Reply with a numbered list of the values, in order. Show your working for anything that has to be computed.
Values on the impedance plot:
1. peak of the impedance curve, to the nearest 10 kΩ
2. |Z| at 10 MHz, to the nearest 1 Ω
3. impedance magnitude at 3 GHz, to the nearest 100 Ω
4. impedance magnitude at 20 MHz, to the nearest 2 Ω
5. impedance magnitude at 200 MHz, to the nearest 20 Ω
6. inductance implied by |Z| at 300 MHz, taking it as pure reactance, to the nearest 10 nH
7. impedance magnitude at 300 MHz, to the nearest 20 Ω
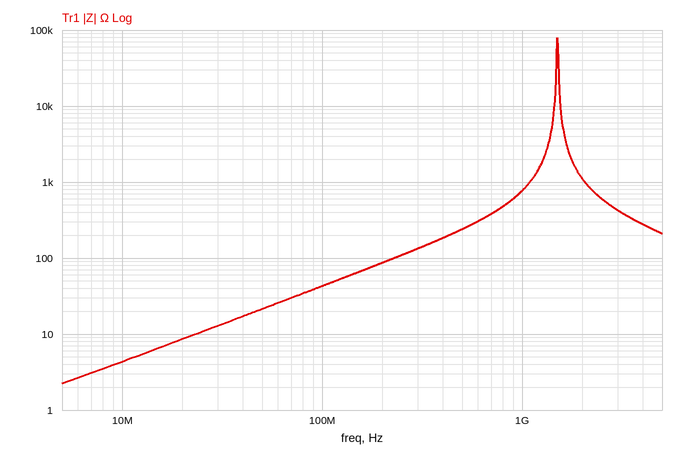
1. 80 kΩ
2. 4 Ω
3. 400 Ω
4. 8 Ω
5. 80 Ω
6. L = 140 Ω/(2π × 300 MHz) ≈ 74.3 nH, so 70 nH to the nearest 10 nH
7. 140 Ω
